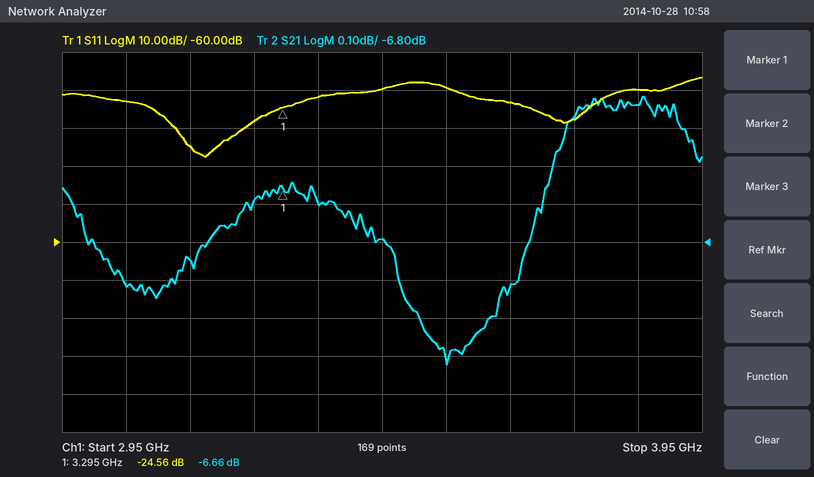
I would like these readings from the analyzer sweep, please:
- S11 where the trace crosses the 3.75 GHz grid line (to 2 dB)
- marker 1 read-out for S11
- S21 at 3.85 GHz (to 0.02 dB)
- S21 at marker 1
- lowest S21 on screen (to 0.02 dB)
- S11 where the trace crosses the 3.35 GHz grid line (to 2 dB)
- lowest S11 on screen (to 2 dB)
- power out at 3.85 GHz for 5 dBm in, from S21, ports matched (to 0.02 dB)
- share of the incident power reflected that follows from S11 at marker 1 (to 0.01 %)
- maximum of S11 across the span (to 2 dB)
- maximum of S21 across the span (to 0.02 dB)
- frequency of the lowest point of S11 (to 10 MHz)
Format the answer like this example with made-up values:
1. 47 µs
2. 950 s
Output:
1. -28 dB
2. -24.56 dB
3. -6.44 dB
4. -6.66 dB
5. -7.12 dB
6. -22 dB
7. -38 dB
8. -1.44 dBm
9. 0.35 %
10. -16 dB
11. -6.42 dB
12. 3.17 GHz
